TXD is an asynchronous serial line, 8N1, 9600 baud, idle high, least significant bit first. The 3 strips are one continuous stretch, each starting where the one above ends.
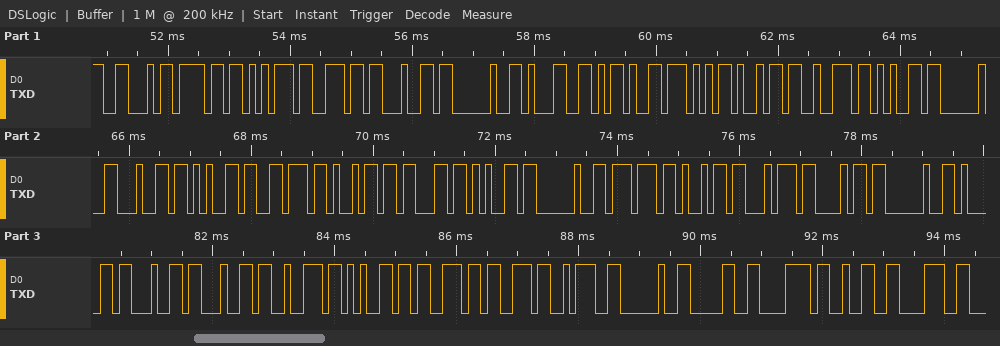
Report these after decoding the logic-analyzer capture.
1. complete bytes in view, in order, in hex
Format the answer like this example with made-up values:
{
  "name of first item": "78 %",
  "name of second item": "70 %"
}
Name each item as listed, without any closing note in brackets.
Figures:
{
  "complete bytes in view, in order, in hex": "46 6F 75 6E 64 20 31 2D 57 69 72 65 20 64 65 76 69 63 65 20 77 69 74 68 20 61 64 64 72 65 73 73 3A 20 30 78 32 38"
}
